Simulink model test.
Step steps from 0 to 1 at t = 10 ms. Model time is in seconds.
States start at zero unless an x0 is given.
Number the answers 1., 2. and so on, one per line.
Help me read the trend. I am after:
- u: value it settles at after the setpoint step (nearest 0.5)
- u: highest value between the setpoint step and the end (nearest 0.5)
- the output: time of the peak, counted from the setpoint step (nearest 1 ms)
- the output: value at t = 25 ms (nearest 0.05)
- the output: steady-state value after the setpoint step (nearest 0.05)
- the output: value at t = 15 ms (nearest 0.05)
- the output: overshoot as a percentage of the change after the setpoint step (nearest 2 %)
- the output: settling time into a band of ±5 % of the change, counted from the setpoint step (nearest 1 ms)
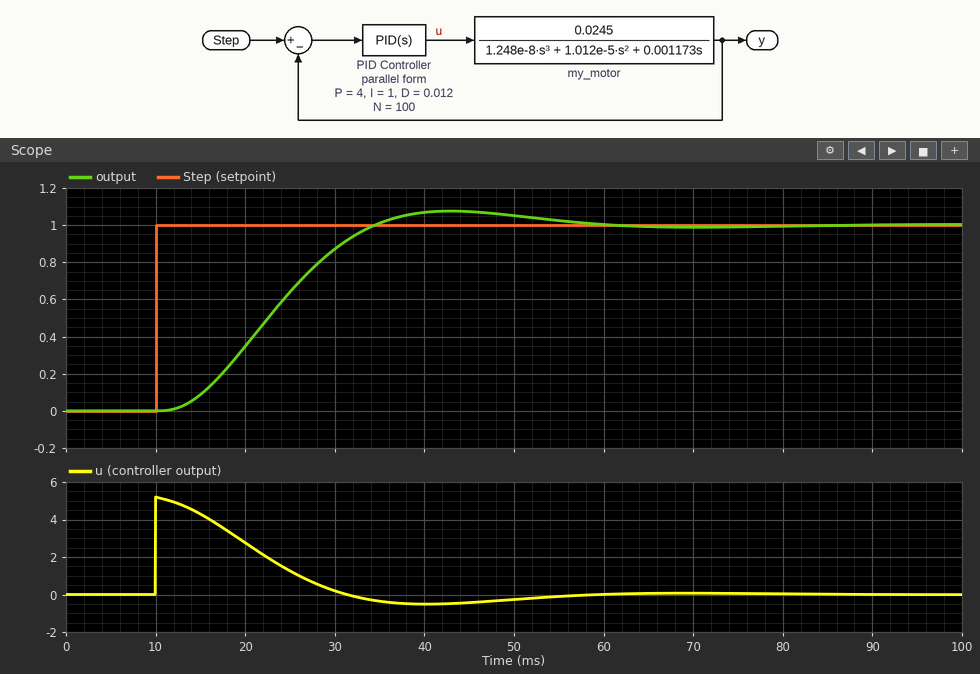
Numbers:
1. 0.0
2. 5.0
3. 33 ms
4. 0.65
5. 1.00
6. 0.10
7. 8 %
8. 40 ms
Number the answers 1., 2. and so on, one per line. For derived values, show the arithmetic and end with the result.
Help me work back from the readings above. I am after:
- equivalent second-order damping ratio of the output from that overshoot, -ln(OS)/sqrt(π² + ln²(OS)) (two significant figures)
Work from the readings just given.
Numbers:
1. ln(0.08) = -2.526; 2.526 / sqrt(9.870 + 6.379) = 0.63
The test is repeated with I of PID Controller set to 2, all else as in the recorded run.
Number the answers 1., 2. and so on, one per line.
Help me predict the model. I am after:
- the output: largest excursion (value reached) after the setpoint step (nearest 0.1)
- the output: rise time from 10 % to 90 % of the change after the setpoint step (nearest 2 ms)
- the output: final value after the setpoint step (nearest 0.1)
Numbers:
1. 1.1
2. 16 ms
3. 1.0
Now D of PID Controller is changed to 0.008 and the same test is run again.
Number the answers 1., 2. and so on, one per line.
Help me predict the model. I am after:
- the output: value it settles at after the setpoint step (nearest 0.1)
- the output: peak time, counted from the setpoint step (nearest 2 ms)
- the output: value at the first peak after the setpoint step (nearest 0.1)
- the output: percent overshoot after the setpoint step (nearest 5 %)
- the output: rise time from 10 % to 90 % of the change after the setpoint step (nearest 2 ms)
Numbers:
1. 1.0
2. 34 ms
3. 1.1
4. 10 %
5. 16 ms
